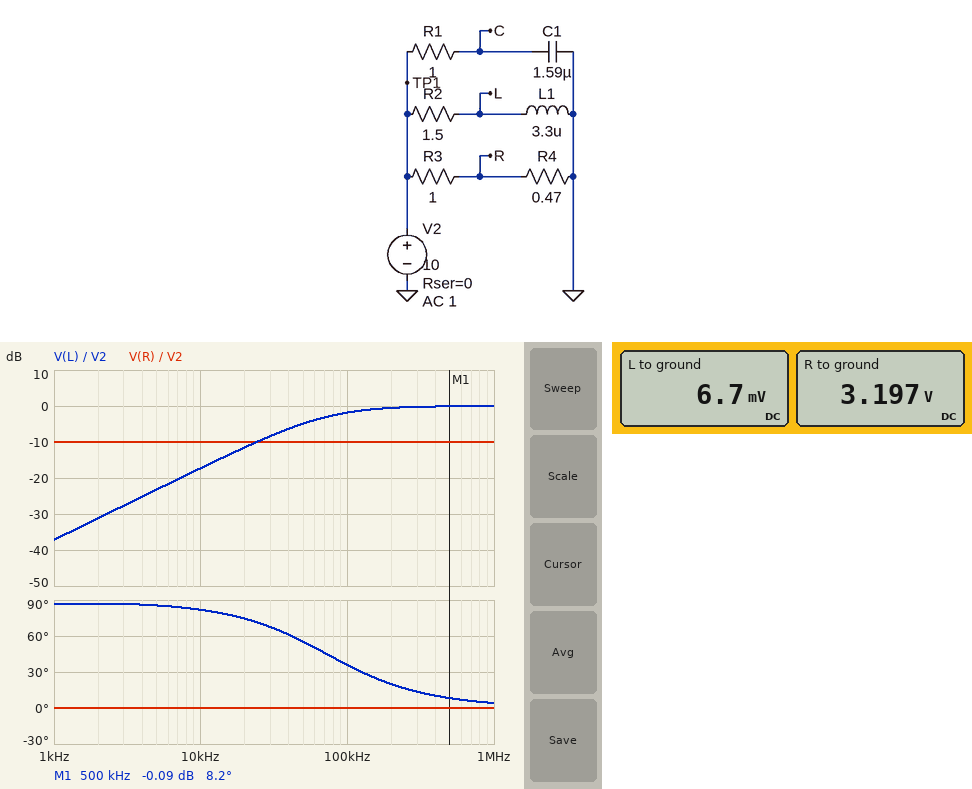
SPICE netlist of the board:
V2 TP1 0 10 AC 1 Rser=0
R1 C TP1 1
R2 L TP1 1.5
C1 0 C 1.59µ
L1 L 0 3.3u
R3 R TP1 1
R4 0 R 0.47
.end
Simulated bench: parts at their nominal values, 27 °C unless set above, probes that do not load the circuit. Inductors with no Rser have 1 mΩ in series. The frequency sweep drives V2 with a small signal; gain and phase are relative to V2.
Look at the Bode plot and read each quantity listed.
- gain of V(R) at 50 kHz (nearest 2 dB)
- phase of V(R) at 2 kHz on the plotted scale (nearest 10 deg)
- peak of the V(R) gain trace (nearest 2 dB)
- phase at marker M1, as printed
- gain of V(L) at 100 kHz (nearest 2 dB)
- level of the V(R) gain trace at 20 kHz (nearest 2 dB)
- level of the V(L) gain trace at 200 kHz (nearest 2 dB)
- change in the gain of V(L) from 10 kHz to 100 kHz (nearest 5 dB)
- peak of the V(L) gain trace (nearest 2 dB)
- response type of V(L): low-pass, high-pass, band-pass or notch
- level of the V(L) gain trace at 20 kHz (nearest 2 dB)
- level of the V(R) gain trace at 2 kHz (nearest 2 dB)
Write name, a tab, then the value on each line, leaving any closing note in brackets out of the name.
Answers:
gain of V(R) at 50 kHz	-10 dB
phase of V(R) at 2 kHz on the plotted scale	0 deg
peak of the V(R) gain trace	-10 dB
phase at marker M1, as printed	8.2 deg
gain of V(L) at 100 kHz	-2 dB
level of the V(R) gain trace at 20 kHz	-10 dB
level of the V(L) gain trace at 200 kHz	0 dB
change in the gain of V(L) from 10 kHz to 100 kHz	15 dB
peak of the V(L) gain trace	0 dB
response type of V(L): low-pass, high-pass, band-pass or notch	high-pass
level of the V(L) gain trace at 20 kHz	-12 dB
level of the V(R) gain trace at 2 kHz	-10 dB
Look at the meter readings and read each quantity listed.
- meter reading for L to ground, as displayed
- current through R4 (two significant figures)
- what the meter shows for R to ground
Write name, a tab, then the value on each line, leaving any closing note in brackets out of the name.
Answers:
meter reading for L to ground, as displayed	6.7 mV
current through R4	6.8 A
what the meter shows for R to ground	3.197 V
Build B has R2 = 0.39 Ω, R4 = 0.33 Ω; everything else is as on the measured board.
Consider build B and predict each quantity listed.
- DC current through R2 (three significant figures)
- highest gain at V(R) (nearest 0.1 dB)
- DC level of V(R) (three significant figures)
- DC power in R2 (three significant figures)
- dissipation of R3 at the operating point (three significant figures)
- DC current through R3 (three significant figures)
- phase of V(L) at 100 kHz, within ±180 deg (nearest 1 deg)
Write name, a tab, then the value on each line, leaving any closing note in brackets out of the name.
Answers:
DC current through R2	25.6 A
highest gain at V(R)	-12.1 dB
DC level of V(R)	2.48 V
DC power in R2	255 W
dissipation of R3 at the operating point	56.5 W
DC current through R3	7.52 A
phase of V(L) at 100 kHz, within ±180 deg	11 deg
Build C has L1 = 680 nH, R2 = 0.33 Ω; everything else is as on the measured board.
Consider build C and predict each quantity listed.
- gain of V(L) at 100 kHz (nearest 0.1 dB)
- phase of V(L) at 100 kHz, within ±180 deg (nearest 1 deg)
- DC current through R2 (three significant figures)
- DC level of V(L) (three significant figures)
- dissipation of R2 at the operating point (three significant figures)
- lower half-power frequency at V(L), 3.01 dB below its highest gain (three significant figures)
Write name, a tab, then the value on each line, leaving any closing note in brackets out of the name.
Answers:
gain of V(L) at 100 kHz	-2.0 dB
phase of V(L) at 100 kHz, within ±180 deg	38 deg
DC current through R2	30.2 A
DC level of V(L)	30.2 mV
dissipation of R2 at the operating point	301 W
lower half-power frequency at V(L), 3.01 dB below its highest gain	77.5 kHz
